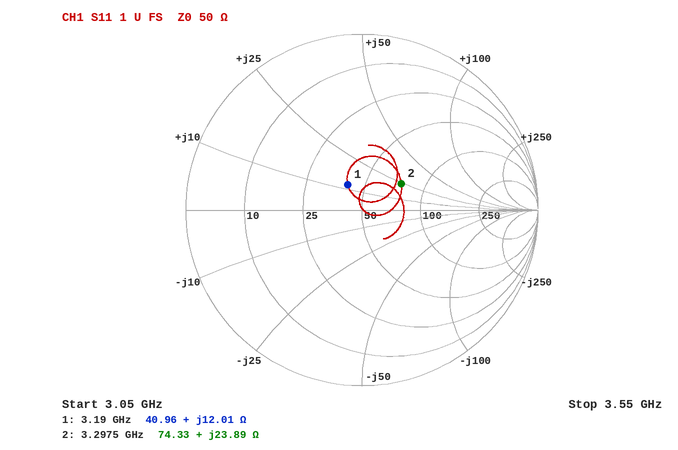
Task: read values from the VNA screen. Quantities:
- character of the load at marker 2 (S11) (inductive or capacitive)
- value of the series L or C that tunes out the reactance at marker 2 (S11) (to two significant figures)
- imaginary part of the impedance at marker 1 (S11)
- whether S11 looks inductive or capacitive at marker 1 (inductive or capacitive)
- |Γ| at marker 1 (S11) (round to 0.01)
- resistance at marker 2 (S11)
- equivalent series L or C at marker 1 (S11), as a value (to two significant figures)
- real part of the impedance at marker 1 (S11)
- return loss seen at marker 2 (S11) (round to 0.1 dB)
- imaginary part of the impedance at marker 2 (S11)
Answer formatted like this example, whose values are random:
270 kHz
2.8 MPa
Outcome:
inductive
2.0 pF
+12.01 Ω
inductive
0.16
74.33 Ω
600 pH
40.96 Ω
11.4 dB
+23.89 Ω
